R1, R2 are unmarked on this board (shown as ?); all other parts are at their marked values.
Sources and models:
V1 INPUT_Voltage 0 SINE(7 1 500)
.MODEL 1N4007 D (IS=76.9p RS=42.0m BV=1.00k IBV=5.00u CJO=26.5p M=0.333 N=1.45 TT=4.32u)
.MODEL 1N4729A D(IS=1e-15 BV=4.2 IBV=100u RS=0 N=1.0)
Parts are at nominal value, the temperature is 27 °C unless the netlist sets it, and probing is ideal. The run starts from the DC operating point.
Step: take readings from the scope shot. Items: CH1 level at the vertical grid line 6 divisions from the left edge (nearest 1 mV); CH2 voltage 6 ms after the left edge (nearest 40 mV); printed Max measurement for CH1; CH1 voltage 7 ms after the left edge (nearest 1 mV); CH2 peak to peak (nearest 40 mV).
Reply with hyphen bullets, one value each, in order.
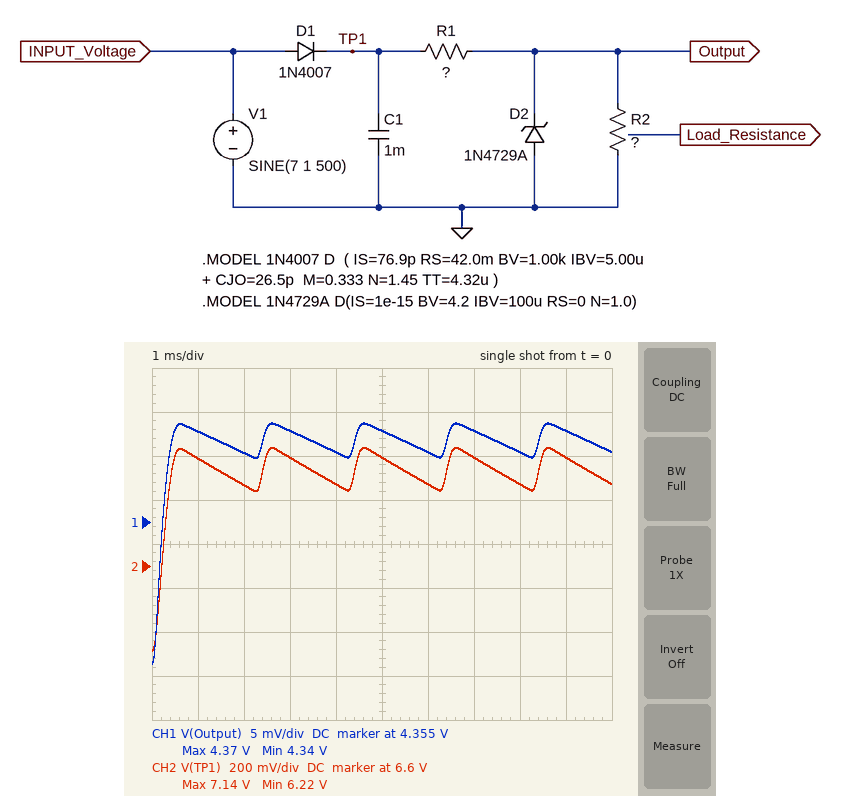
- 4.363 V
- 6.96 V
- 4.37 V
- 4.365 V
- 920 mV
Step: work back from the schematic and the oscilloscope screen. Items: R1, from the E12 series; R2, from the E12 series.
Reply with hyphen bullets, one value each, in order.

- 22 Ω
- 68 Ω
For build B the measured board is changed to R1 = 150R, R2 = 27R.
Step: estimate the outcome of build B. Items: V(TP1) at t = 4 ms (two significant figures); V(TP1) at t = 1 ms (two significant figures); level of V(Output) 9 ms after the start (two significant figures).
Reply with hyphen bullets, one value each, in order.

- 7.1 V
- 7.1 V
- 1.1 V
